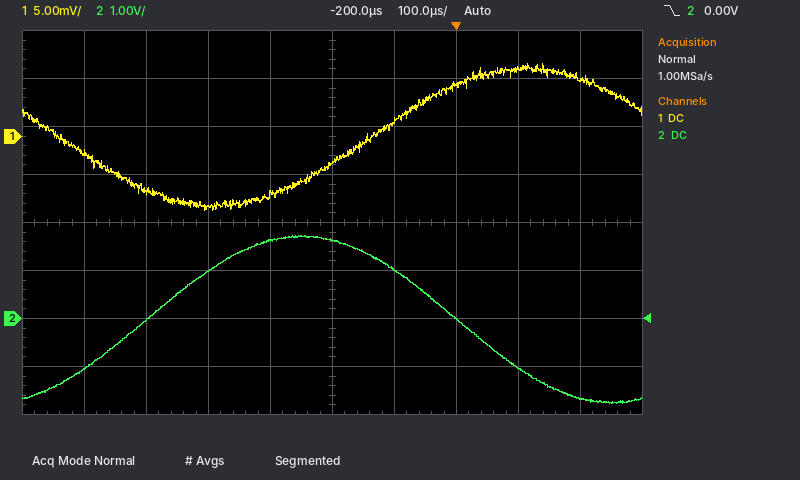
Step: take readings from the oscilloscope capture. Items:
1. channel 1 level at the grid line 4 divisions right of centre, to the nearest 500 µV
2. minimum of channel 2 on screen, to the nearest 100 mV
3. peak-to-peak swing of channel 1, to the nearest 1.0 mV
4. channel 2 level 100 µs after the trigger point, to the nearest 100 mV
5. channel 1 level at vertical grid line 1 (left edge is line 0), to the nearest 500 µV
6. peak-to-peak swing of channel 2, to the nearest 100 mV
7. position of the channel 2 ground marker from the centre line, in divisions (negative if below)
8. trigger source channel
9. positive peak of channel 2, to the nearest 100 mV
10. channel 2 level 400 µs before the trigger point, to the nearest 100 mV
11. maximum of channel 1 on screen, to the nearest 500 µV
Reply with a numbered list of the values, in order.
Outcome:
1. 6.0 mV
2. -1.8 V
3. 15.0 mV
4. -1.0 V
5. -1.5 mV
6. 3.5 V
7. -2.0 div
8. channel 2
9. 1.7 V
10. 1.0 V
11. 7.5 mV
